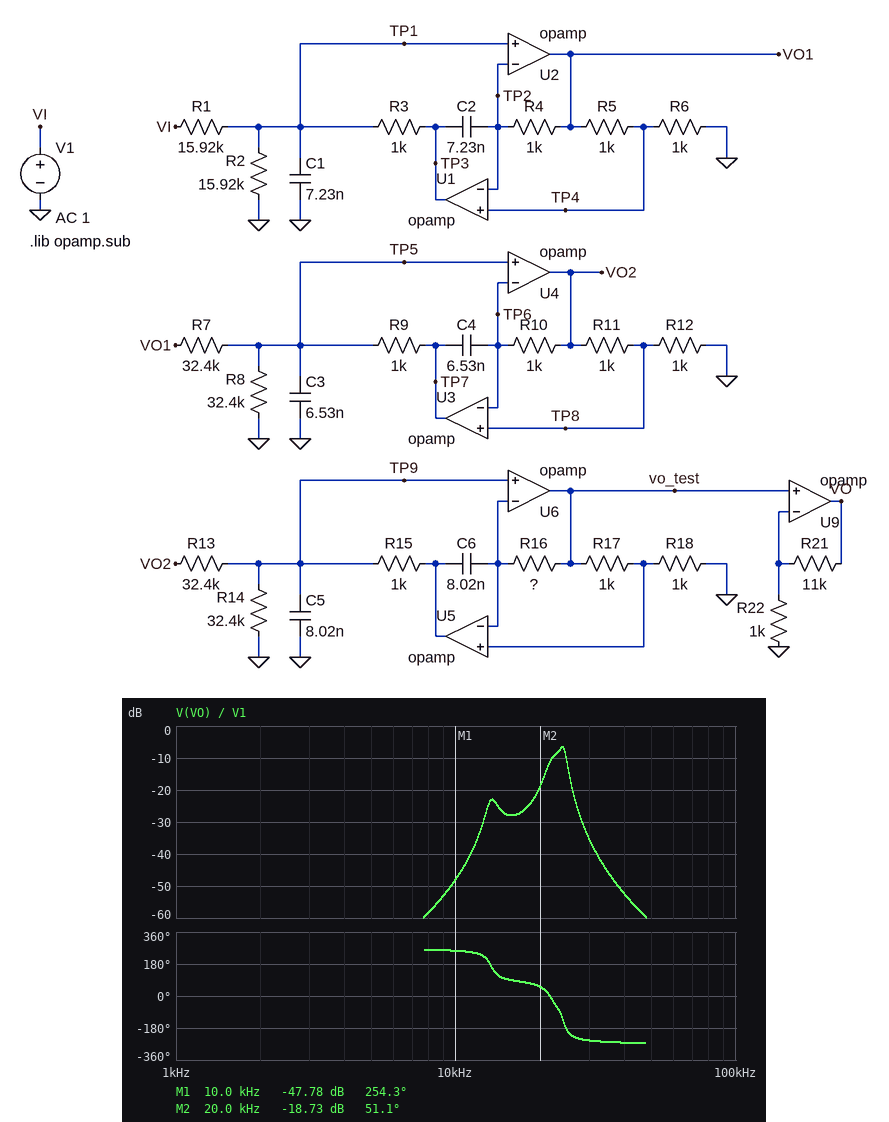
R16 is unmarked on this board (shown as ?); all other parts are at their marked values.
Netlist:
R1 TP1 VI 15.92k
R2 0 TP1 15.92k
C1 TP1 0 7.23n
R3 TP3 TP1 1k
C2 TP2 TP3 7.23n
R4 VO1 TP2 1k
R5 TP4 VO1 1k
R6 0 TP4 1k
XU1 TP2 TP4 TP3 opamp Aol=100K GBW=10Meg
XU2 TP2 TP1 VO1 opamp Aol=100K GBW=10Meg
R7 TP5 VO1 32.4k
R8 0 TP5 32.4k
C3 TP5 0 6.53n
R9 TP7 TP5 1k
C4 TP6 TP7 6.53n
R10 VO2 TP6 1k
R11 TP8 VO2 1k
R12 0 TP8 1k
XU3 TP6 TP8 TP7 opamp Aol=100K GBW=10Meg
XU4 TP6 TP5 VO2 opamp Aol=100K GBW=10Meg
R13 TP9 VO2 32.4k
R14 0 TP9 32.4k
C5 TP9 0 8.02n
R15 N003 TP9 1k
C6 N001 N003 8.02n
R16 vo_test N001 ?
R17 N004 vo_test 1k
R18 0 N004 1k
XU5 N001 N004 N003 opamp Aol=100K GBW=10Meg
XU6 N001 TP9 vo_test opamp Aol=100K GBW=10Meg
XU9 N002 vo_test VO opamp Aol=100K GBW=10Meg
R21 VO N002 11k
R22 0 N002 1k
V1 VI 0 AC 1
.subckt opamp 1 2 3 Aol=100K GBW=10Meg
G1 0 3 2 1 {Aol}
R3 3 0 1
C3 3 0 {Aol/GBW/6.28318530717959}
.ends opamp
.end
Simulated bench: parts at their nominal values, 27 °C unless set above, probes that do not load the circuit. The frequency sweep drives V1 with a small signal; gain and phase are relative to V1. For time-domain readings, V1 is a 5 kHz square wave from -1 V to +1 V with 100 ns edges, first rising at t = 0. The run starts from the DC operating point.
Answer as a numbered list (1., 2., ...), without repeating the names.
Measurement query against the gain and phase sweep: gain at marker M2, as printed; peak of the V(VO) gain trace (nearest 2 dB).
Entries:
1. -18.73 dB
2. -6 dB
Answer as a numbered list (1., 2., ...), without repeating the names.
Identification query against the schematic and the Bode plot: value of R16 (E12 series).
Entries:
1. 2.2 kΩ
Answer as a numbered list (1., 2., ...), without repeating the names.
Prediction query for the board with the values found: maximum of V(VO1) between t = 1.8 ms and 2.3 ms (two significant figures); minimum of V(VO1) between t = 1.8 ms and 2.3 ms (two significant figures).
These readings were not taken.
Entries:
1. 180 mV
2. -180 mV
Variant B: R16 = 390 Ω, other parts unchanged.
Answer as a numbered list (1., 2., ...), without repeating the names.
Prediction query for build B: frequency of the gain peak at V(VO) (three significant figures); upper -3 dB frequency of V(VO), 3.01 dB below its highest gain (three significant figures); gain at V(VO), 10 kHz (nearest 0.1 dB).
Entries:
1. 24.2 kHz
2. 24.9 kHz
3. -68.9 dB
